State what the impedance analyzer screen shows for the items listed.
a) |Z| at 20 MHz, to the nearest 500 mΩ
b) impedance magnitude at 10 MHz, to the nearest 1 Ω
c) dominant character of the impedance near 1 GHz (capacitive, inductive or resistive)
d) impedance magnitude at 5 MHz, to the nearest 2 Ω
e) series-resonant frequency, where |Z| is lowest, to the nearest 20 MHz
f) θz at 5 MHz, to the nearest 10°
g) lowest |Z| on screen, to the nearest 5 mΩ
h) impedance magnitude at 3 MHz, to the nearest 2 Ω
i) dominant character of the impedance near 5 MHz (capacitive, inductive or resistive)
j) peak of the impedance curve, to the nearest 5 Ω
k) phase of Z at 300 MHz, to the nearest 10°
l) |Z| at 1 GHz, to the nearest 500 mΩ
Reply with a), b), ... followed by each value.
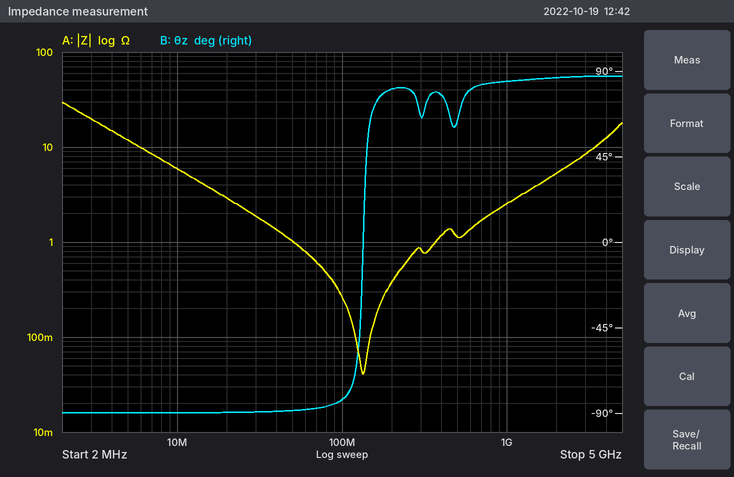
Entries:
a) 3.0 Ω
b) 6 Ω
c) inductive
d) 12 Ω
e) 140 MHz
f) -90°
g) 40 mΩ
h) 20 Ω
i) capacitive
j) 30 Ω
k) 70°
l) 2.5 Ω
